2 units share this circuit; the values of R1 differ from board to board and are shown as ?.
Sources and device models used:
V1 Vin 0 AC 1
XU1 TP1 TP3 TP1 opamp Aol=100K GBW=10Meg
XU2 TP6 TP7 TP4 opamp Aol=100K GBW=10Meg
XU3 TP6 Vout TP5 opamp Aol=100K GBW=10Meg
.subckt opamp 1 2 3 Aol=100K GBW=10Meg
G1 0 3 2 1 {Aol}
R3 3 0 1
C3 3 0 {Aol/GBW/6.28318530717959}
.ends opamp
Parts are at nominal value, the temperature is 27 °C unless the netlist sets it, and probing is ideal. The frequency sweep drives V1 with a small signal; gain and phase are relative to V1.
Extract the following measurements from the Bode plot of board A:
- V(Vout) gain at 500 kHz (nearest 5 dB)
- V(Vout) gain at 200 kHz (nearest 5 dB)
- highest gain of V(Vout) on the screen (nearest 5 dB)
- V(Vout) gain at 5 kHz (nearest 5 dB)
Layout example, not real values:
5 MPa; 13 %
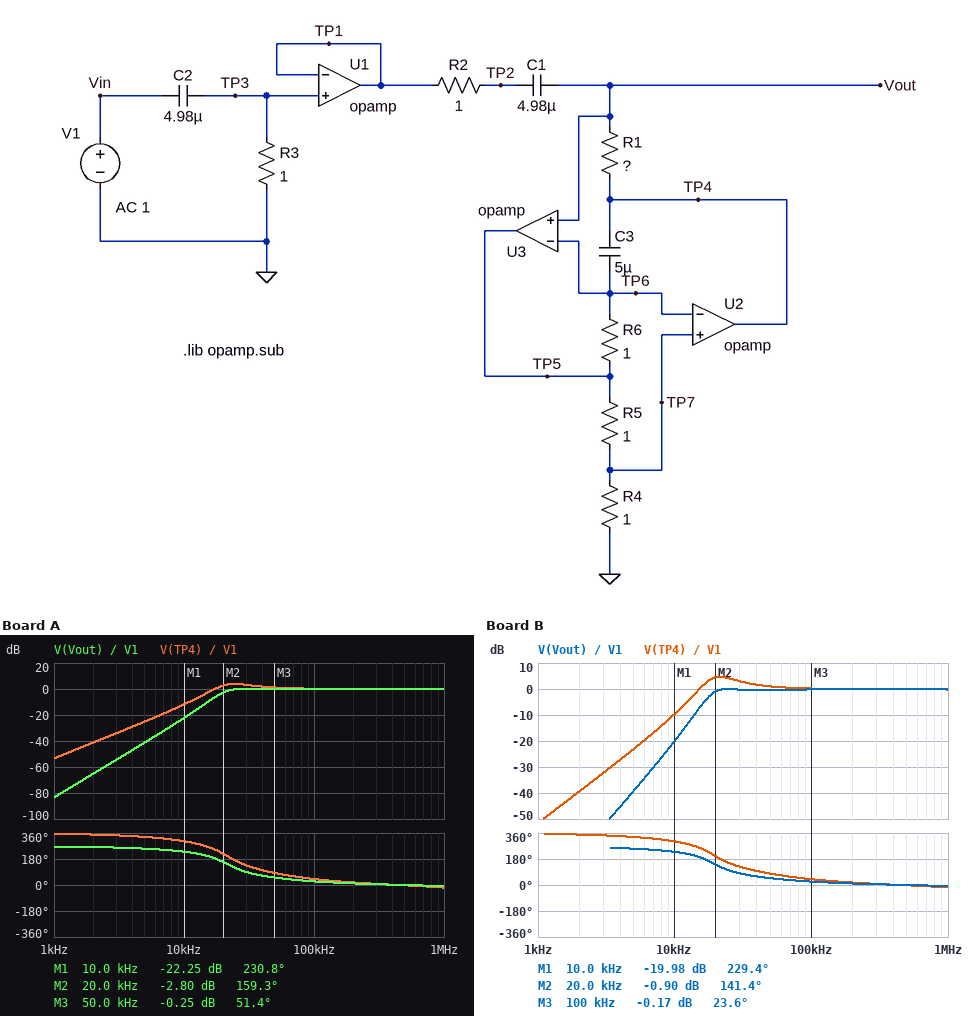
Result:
0 dB; 0 dB; 0 dB; -40 dB
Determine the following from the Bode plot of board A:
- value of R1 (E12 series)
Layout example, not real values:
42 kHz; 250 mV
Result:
2.2 Ω
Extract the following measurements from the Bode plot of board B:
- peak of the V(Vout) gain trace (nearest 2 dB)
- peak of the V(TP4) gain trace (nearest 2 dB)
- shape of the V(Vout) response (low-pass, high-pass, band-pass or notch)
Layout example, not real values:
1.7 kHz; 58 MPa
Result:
0 dB; 4 dB; high-pass
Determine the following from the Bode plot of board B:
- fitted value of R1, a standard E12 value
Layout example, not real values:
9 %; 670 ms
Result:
2.7 Ω
